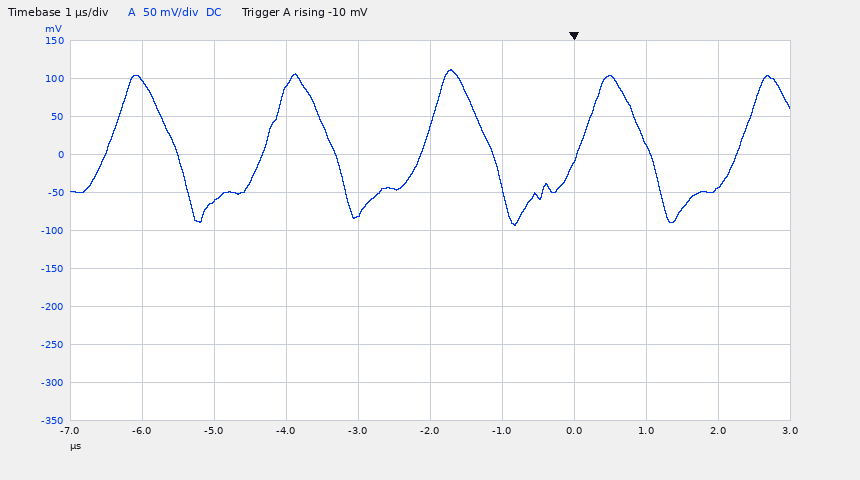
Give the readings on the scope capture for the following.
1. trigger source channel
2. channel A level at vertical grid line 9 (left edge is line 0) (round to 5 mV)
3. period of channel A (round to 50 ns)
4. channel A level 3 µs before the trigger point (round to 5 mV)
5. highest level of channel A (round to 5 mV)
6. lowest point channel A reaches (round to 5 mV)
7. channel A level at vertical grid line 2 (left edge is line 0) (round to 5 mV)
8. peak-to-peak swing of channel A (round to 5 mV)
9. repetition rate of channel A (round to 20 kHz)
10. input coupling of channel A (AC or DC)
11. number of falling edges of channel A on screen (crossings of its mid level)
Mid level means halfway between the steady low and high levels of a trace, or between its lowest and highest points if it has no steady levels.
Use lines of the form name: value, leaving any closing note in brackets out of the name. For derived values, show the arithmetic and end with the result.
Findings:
trigger source channel: channel A
channel A level at vertical grid line 9 (left edge is line 0): -45 mV
period of channel A: 2.20 µs
channel A level 3 µs before the trigger point: -80 mV
highest level of channel A: 110 mV
lowest point channel A reaches: -95 mV
channel A level at vertical grid line 2 (left edge is line 0): -60 mV
peak-to-peak swing of channel A: 110 mV − (-95 mV) = 205 mV
repetition rate of channel A: 1 / 2.20 µs ≈ 455 kHz, so 460 kHz to the nearest 20 kHz
input coupling of channel A: DC
number of falling edges of channel A on screen: 4
